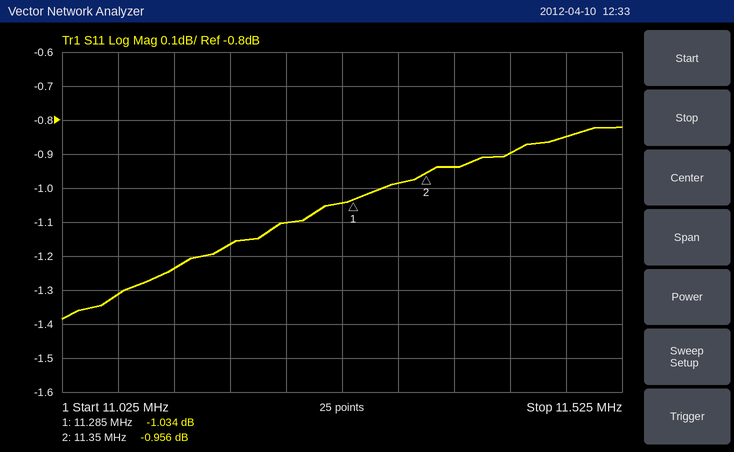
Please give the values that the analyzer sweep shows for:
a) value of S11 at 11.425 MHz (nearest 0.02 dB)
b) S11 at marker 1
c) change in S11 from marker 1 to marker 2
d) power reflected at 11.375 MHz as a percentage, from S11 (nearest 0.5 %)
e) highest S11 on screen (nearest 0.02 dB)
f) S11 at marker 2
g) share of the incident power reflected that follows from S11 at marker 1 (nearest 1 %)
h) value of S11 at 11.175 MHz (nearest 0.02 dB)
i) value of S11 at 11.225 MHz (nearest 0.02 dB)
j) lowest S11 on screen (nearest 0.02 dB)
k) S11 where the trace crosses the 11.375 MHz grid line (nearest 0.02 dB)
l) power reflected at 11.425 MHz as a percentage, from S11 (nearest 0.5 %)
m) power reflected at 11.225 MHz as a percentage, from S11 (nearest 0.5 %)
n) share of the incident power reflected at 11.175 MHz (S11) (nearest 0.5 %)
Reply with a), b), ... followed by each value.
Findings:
a) -0.90 dB
b) -1.034 dB
c) 0.078 dB
d) 80.5 %
e) -0.82 dB
f) -0.956 dB
g) 79 %
h) -1.16 dB
i) -1.10 dB
j) -1.38 dB
k) -0.94 dB
l) 81.5 %
m) 77.5 %
n) 76.5 %
